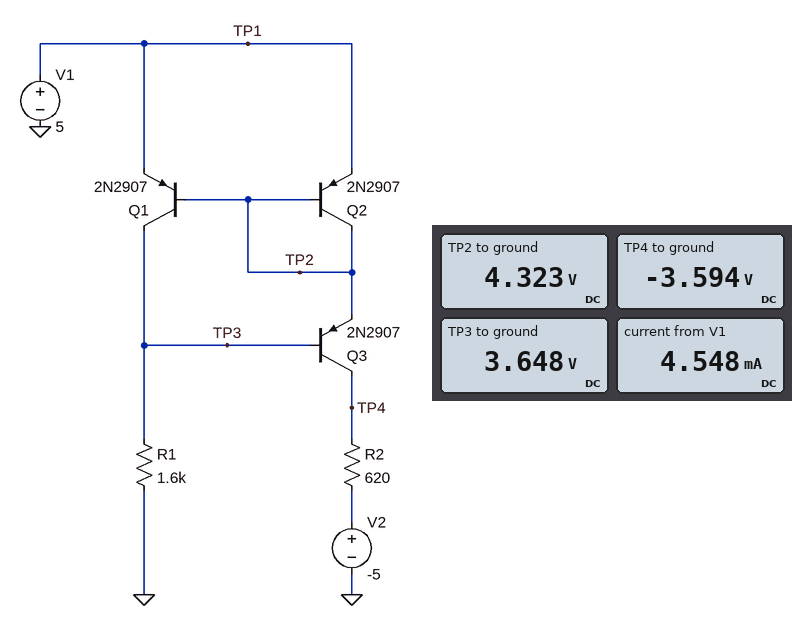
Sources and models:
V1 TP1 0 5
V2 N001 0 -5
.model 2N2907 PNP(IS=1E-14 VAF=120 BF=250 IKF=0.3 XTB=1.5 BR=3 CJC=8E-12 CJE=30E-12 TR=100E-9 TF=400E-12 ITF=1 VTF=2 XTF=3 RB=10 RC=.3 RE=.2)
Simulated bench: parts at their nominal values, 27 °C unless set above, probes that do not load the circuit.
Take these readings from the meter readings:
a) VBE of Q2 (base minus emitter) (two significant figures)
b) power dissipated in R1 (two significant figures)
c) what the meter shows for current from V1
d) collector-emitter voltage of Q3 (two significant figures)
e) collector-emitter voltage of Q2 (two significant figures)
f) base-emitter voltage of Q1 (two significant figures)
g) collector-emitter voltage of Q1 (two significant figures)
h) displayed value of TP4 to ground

-680 mV
8.3 mW
4.548 mA
-7.9 V
-680 mV
-680 mV
-1.4 V
-3.594 V
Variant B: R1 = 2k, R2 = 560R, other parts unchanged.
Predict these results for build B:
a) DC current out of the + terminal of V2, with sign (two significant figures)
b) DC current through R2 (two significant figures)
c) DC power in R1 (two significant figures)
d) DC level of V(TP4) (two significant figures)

-1.8 mA
1.8 mA
6.7 mW
-4.0 V
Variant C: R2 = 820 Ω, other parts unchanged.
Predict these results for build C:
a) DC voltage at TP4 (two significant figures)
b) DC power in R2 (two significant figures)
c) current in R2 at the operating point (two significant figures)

-3.1 V
4.2 mW
2.3 mA
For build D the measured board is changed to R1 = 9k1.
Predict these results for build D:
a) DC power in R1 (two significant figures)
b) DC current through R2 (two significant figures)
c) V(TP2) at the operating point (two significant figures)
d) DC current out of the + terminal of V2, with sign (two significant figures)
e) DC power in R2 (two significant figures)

1.5 mW
410 µA
4.4 V
-410 µA
100 µW
